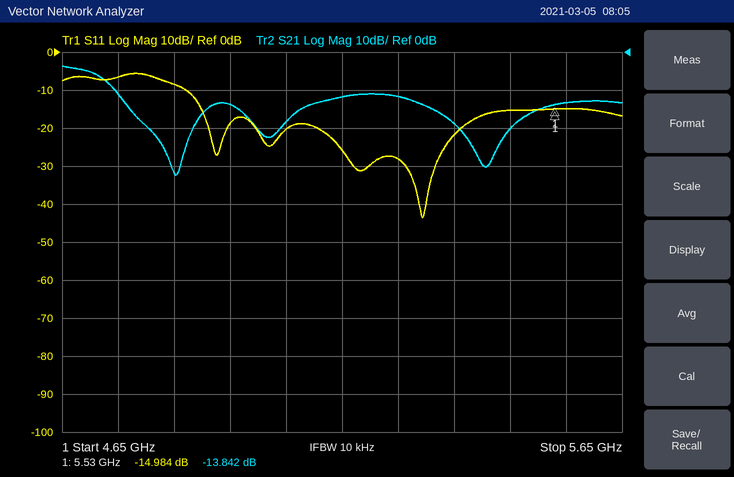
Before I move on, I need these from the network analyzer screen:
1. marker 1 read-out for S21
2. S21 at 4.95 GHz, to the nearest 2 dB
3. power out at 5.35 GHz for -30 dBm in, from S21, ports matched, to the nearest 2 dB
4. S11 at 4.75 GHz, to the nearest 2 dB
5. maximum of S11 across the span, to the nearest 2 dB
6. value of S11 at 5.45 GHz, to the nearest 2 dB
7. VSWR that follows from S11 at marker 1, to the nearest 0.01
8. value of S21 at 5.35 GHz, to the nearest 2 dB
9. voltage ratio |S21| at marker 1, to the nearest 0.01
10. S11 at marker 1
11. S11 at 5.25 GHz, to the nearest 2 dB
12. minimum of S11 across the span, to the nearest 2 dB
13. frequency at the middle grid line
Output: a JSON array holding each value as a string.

["-13.842 dB", "-14 dB", "-48 dBm", "-6 dB", "-6 dB", "-16 dB", "1.43", "-18 dB", "0.20", "-14.984 dB", "-28 dB", "-44 dB", "5.15 GHz"]
